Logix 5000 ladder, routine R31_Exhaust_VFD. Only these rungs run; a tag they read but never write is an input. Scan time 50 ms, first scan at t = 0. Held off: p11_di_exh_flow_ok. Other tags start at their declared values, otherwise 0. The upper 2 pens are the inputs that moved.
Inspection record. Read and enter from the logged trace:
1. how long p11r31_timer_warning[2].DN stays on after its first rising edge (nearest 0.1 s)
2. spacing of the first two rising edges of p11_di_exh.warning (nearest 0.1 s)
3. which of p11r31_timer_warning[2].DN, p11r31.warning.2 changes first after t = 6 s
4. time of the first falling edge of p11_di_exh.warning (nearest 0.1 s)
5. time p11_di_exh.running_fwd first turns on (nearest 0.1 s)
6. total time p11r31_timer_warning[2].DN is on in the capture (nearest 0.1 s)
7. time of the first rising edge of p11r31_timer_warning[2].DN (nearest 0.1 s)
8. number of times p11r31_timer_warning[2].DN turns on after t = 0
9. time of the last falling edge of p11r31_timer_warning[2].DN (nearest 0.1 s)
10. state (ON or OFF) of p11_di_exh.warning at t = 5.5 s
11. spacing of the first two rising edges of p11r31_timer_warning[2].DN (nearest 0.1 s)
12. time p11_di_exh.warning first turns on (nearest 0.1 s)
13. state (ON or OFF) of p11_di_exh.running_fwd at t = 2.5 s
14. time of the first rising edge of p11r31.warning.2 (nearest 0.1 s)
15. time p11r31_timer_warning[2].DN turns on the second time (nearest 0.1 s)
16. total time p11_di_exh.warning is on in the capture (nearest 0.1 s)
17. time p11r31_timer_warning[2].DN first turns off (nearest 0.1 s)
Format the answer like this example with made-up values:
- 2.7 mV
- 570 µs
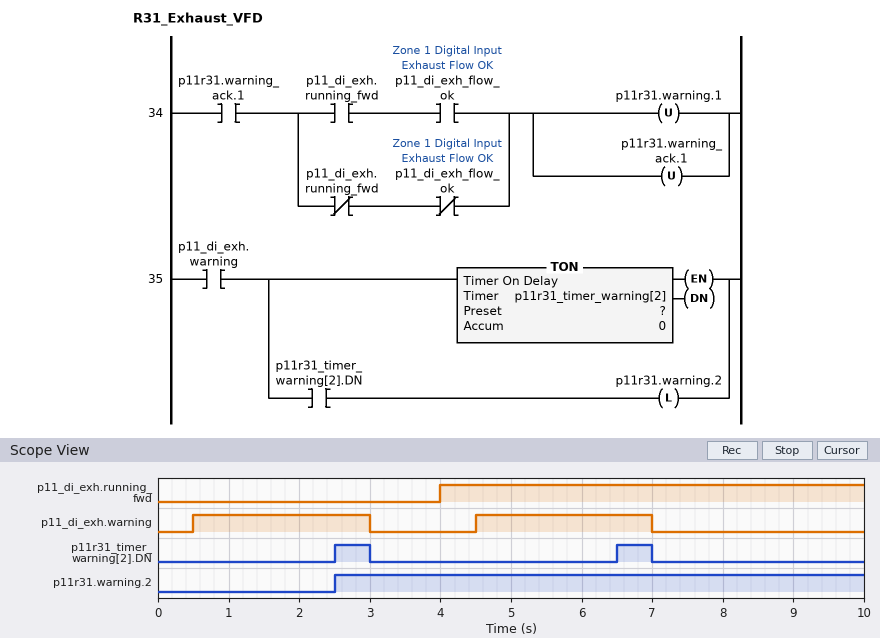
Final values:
- 0.5 s
- 4.0 s
- p11r31_timer_warning[2].DN
- 3.0 s
- 4.0 s
- 1.0 s
- 2.5 s
- 2
- 7.0 s
- ON
- 4.0 s
- 0.5 s
- OFF
- 2.5 s
- 6.5 s
- 5.0 s
- 3.0 s
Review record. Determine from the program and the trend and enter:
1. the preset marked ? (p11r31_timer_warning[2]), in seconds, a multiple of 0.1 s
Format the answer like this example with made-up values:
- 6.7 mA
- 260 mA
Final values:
- 2.0 s
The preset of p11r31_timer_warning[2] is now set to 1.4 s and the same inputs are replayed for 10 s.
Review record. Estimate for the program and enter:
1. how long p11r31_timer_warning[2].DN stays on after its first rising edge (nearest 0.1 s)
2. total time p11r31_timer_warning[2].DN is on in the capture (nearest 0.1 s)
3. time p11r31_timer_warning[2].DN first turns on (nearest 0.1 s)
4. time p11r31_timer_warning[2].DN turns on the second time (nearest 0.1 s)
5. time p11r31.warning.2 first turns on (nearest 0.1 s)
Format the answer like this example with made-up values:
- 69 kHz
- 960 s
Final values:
- 1.1 s
- 2.2 s
- 1.9 s
- 5.9 s
- 1.9 s
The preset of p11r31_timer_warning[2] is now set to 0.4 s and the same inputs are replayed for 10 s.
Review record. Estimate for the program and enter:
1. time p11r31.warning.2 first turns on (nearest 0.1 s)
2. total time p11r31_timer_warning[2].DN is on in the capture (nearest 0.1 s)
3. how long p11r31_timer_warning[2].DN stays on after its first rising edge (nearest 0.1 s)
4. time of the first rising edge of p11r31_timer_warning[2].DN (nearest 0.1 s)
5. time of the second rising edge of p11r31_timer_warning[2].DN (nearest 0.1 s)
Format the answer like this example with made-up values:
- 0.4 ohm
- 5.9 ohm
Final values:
- 0.9 s
- 4.2 s
- 2.1 s
- 0.9 s
- 4.9 s
